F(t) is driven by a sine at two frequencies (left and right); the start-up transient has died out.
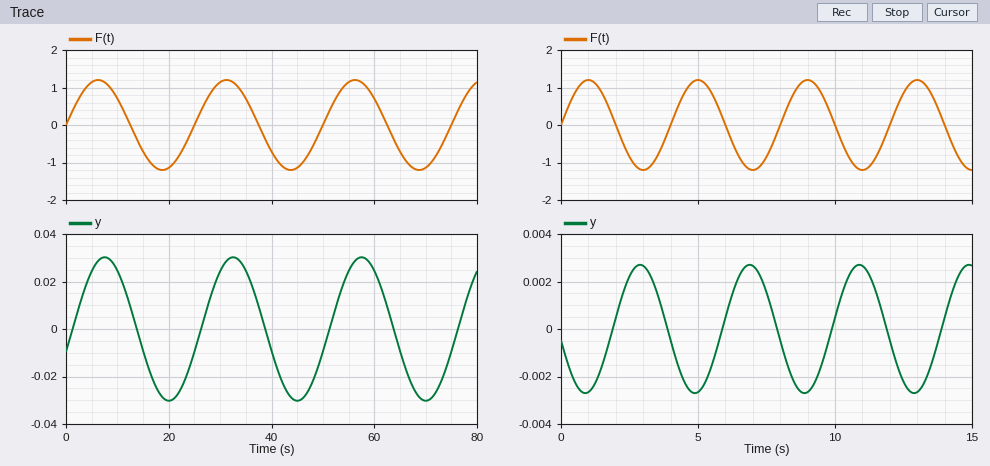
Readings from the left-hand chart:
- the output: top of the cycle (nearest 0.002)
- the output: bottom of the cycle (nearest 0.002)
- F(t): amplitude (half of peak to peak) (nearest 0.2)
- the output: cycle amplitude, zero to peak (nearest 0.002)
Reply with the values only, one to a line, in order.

0.030
-0.030
1.2
0.030
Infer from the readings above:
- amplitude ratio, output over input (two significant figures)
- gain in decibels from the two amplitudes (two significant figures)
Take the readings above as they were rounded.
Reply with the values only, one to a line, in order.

0.025
-32 dB
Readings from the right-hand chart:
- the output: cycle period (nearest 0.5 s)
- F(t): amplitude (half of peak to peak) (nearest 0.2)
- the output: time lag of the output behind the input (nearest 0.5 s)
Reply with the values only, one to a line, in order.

4.0 s
1.2
2.0 s
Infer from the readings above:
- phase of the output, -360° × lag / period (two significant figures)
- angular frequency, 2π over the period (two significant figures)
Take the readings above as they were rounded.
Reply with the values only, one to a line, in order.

-180°
1.6 rad/s
